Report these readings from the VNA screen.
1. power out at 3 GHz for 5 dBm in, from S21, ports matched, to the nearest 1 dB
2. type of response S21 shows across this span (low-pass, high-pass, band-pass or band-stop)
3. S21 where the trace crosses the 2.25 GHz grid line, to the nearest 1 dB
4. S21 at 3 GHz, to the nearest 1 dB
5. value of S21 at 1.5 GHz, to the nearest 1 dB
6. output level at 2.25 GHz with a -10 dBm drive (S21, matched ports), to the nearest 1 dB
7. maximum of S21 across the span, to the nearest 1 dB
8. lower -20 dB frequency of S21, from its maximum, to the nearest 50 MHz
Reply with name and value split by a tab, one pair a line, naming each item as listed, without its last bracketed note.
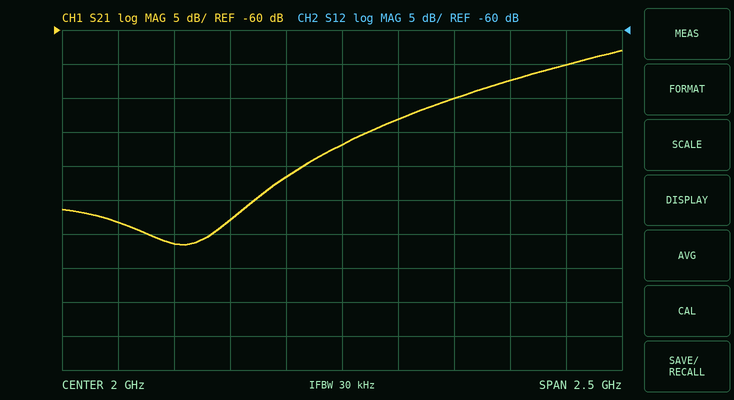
power out at 3 GHz for 5 dBm in, from S21, ports matched, to the nearest 1 dB	-60 dBm
type of response S21 shows across this span	high-pass
S21 where the trace crosses the 2.25 GHz grid line, to the nearest 1 dB	-73 dB
S21 at 3 GHz, to the nearest 1 dB	-65 dB
value of S21 at 1.5 GHz, to the nearest 1 dB	-88 dB
output level at 2.25 GHz with a -10 dBm drive (S21, matched ports), to the nearest 1 dB	-83 dBm
maximum of S21 across the span, to the nearest 1 dB	-63 dB
lower -20 dB frequency of S21, from its maximum, to the nearest 50 MHz	1.70 GHz
